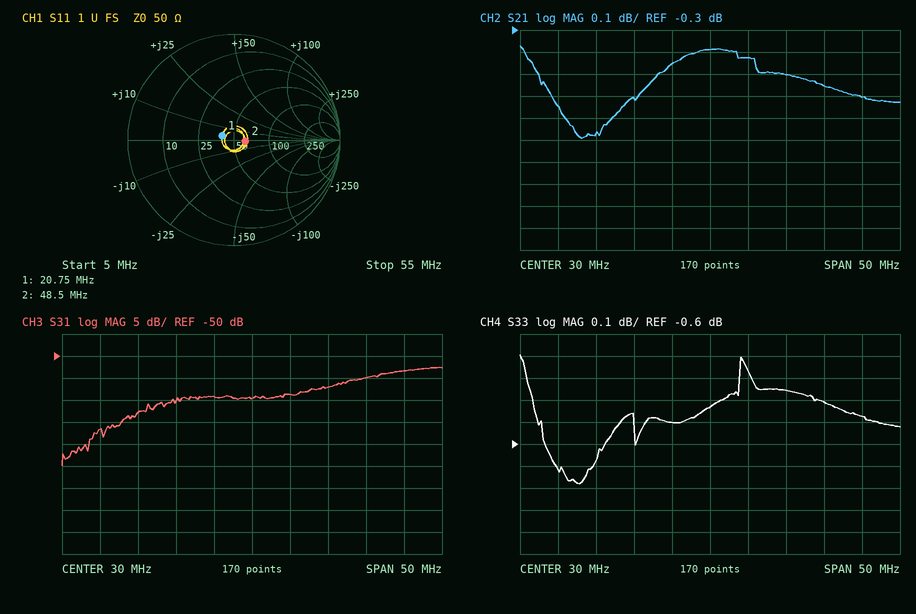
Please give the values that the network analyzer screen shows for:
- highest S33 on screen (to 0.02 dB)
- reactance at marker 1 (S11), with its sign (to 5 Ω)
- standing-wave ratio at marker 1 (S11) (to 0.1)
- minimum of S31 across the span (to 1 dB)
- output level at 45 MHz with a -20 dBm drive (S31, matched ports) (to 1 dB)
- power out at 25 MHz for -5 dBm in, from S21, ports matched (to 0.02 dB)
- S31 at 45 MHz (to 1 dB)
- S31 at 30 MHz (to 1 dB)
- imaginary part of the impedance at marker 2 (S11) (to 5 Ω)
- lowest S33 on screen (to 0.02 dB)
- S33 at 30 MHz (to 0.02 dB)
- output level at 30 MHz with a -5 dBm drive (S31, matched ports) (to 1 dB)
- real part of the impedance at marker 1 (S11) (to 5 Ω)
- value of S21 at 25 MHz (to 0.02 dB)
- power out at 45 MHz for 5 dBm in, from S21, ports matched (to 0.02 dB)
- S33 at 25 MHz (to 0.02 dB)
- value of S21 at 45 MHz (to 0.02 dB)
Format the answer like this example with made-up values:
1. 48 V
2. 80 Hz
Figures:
1. -0.20 dB
2. +5 Ω
3. 1.3
4. -75 dB
5. -75 dBm
6. -5.46 dBm
7. -55 dB
8. -60 dB
9. 0 Ω
10. -0.78 dB
11. -0.44 dB
12. -65 dBm
13. 40 Ω
14. -0.46 dB
15. 4.44 dBm
16. -0.50 dB
17. -0.56 dB
